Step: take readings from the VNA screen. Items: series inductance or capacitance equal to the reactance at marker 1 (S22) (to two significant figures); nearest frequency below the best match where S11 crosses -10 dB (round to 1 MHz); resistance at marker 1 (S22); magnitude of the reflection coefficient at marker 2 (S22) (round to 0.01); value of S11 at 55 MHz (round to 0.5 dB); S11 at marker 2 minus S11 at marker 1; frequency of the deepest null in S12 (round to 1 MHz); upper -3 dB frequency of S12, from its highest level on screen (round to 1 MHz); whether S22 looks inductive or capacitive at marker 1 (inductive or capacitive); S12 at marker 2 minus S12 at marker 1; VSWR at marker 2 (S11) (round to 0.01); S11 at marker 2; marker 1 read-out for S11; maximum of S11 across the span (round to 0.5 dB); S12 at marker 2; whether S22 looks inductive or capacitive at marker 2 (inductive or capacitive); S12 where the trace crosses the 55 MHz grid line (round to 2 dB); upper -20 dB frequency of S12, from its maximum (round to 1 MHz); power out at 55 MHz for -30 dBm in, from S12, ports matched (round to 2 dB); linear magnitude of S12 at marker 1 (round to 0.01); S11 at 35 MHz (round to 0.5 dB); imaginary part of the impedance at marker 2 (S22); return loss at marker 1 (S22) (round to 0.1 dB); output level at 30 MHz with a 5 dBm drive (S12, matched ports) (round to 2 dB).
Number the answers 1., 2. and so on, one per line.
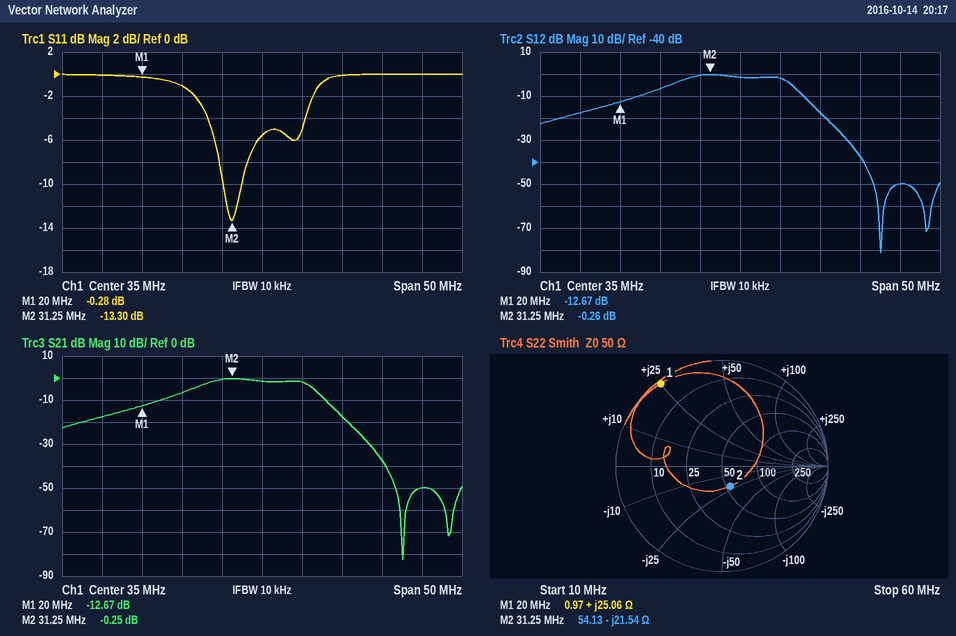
1. 200 nH
2. 30 MHz
3. 0.97 Ω
4. 0.21
5. 0.0 dB
6. -13.02 dB
7. 53 MHz
8. 41 MHz
9. inductive
10. 12.41 dB
11. 1.55
12. -13.30 dB
13. -0.28 dB
14. 0.0 dB
15. -0.26 dB
16. capacitive
17. -50 dB
18. 46 MHz
19. -80 dBm
20. 0.23
21. -5.5 dB
22. -21.54 Ω
23. 0.3 dB
24. 4 dBm
